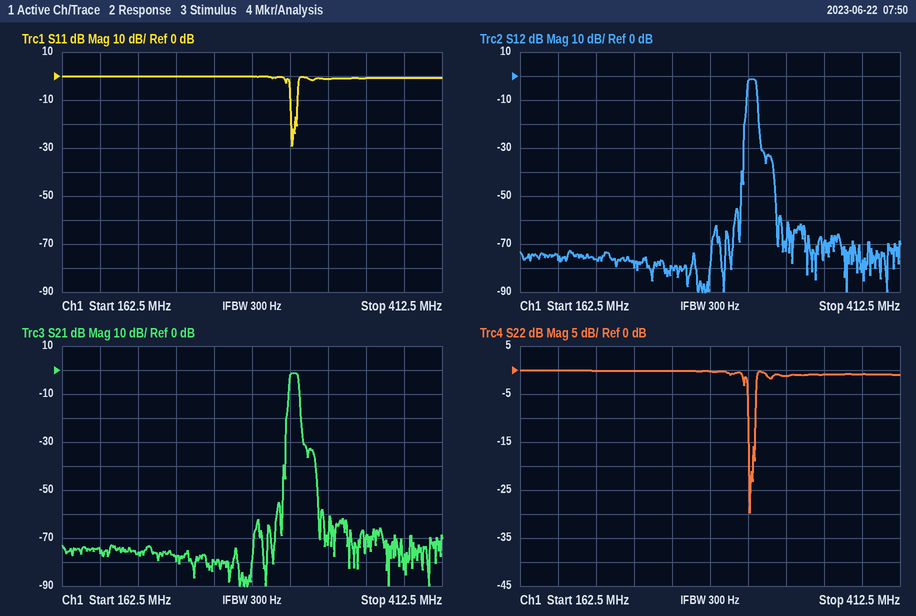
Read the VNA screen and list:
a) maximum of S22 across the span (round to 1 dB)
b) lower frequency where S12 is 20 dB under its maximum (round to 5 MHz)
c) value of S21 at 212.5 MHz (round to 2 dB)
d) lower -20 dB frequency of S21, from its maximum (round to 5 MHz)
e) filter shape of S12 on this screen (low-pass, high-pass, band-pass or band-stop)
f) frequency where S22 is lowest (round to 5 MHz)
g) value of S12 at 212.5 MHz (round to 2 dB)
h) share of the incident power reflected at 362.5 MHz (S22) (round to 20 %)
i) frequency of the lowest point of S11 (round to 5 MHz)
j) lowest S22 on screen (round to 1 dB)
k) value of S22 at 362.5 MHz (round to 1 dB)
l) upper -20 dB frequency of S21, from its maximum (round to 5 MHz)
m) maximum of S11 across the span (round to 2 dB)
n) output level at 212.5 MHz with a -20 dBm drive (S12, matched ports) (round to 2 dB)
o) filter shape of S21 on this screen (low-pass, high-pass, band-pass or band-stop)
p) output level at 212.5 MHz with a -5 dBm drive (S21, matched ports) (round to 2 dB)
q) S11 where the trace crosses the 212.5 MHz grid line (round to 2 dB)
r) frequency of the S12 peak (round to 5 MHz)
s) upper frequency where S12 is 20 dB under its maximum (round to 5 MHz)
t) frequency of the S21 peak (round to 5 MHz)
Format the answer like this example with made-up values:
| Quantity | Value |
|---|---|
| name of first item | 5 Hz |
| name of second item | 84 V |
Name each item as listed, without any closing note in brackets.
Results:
| Quantity | Value |
|---|---|
| maximum of S22 across the span | 0 dB |
| lower frequency where S12 is 20 dB under its maximum | 310 MHz |
| value of S21 at 212.5 MHz | -76 dB |
| lower -20 dB frequency of S21, from its maximum | 310 MHz |
| filter shape of S12 on this screen | band-pass |
| frequency where S22 is lowest | 315 MHz |
| value of S12 at 212.5 MHz | -76 dB |
| share of the incident power reflected at 362.5 MHz (S22) | 80 % |
| frequency of the lowest point of S11 | 315 MHz |
| lowest S22 on screen | -30 dB |
| value of S22 at 362.5 MHz | -1 dB |
| upper -20 dB frequency of S21, from its maximum | 320 MHz |
| maximum of S11 across the span | 0 dB |
| output level at 212.5 MHz with a -20 dBm drive (S12, matched ports) | -96 dBm |
| filter shape of S21 on this screen | band-pass |
| output level at 212.5 MHz with a -5 dBm drive (S21, matched ports) | -82 dBm |
| S11 where the trace crosses the 212.5 MHz grid line | 0 dB |
| frequency of the S12 peak | 315 MHz |
| upper frequency where S12 is 20 dB under its maximum | 320 MHz |
| frequency of the S21 peak | 315 MHz |
